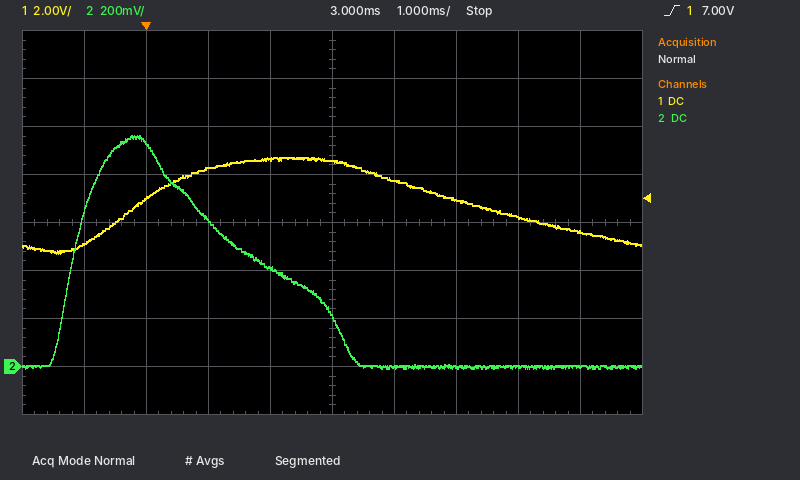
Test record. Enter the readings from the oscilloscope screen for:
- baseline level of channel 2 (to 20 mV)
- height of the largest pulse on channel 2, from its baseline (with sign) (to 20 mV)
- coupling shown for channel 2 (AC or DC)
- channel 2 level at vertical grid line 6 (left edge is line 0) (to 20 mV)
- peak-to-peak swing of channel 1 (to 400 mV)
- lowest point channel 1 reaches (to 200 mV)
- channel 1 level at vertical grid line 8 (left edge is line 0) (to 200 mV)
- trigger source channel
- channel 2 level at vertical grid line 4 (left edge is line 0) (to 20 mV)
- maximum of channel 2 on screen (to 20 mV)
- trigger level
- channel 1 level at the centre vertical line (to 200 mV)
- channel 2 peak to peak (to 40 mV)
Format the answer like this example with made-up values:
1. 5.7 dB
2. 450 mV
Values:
1. 0 mV
2. +960 mV
3. DC
4. 0 mV
5. 4.0 V
6. 4.8 V
7. 6.2 V
8. channel 1
9. 400 mV
10. 960 mV
11. 7.00 V
12. 8.6 V
13. 960 mV
